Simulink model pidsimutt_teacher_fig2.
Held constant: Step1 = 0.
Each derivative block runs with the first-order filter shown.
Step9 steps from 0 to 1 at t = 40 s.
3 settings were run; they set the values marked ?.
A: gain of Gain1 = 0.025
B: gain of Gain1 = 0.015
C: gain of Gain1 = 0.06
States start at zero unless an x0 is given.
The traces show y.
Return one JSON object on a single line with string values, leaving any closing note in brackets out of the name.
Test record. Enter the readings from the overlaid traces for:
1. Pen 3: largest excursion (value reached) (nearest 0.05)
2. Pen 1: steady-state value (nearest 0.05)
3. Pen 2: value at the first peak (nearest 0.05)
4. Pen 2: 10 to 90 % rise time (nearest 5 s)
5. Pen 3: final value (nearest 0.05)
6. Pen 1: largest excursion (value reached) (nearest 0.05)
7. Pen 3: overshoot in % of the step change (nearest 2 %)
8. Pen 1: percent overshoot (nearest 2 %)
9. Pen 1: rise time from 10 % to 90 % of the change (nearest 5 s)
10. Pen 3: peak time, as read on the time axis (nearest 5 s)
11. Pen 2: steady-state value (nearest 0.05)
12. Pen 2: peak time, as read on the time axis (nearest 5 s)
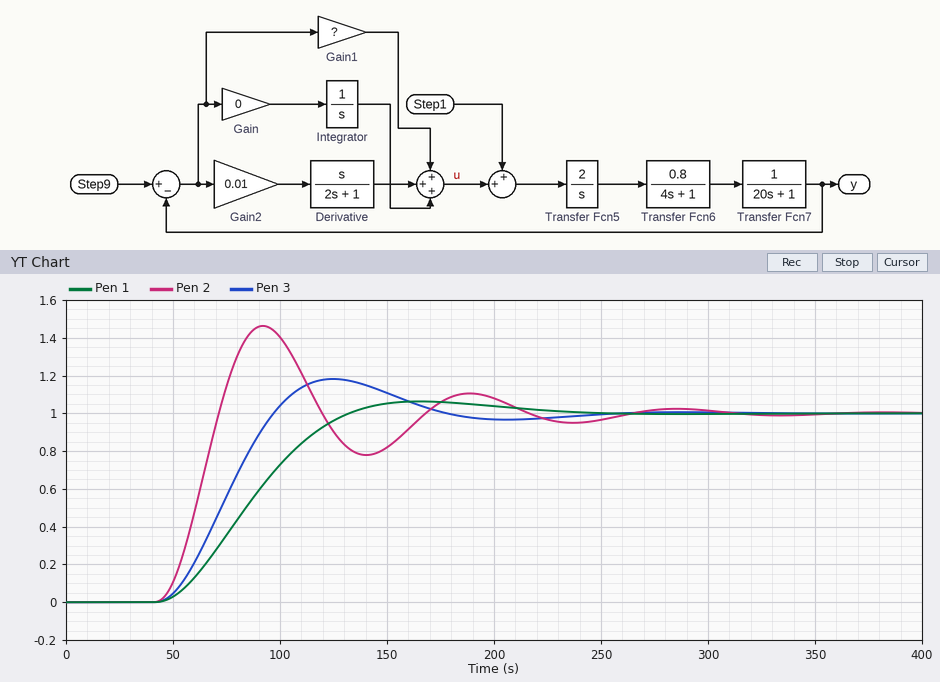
{"Pen 3: largest excursion (value reached)": "1.20", "Pen 1: steady-state value": "1.00", "Pen 2: value at the first peak": "1.45", "Pen 2: 10 to 90 % rise time": "20 s", "Pen 3: final value": "1.00", "Pen 1: largest excursion (value reached)": "1.05", "Pen 3: overshoot in % of the step change": "18 %", "Pen 1: percent overshoot": "6 %", "Pen 1: rise time from 10 % to 90 % of the change": "60 s", "Pen 3: peak time, as read on the time axis": "125 s", "Pen 2: steady-state value": "1.00", "Pen 2: peak time, as read on the time axis": "90 s"}
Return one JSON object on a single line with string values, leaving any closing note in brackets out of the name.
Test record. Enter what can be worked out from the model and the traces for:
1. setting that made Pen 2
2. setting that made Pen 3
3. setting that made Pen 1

{"setting that made Pen 2": "C", "setting that made Pen 3": "A", "setting that made Pen 1": "B"}
